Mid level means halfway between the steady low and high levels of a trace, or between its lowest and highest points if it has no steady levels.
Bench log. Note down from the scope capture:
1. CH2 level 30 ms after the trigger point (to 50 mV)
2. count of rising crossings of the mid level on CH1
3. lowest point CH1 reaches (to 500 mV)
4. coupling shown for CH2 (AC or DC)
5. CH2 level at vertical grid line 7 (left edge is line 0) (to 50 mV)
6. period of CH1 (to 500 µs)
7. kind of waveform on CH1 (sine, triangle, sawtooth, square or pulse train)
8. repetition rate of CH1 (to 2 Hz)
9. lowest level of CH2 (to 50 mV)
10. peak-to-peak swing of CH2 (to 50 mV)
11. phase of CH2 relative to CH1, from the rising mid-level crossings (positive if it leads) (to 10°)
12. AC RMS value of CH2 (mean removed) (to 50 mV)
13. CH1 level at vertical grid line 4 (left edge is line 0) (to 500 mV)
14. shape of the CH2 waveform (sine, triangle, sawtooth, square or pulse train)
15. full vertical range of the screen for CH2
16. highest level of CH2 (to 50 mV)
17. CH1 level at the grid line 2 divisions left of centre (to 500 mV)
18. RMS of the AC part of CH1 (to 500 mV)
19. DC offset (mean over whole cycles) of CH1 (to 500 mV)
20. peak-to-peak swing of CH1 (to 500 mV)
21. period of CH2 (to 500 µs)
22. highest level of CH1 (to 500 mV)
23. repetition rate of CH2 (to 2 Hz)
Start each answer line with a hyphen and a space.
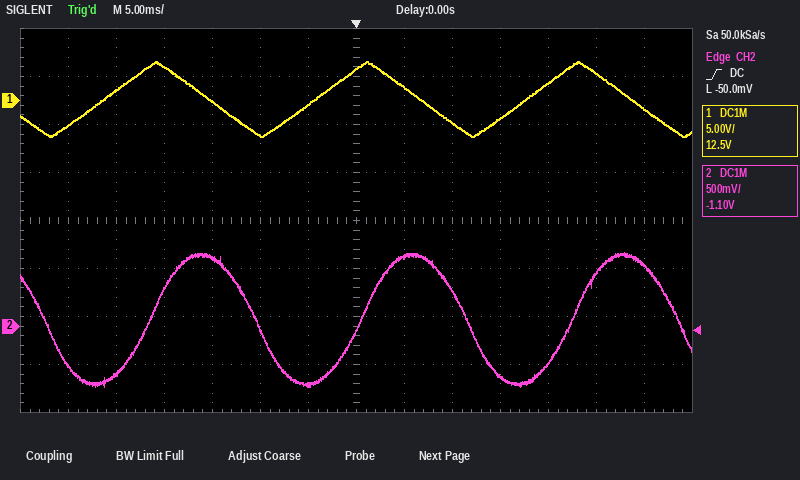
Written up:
- 650 mV
- 3
- -4.0 V
- DC
- -50 mV
- 22.0 ms
- triangle
- 46 Hz
- -650 mV
- 1.40 V
- -80°
- 500 mV
- 0.0 V
- sine
- 4 V
- 750 mV
- -3.5 V
- 2.5 V
- 0.0 V
- 8.0 V
- 22.0 ms
- 4.0 V
- 46 Hz
